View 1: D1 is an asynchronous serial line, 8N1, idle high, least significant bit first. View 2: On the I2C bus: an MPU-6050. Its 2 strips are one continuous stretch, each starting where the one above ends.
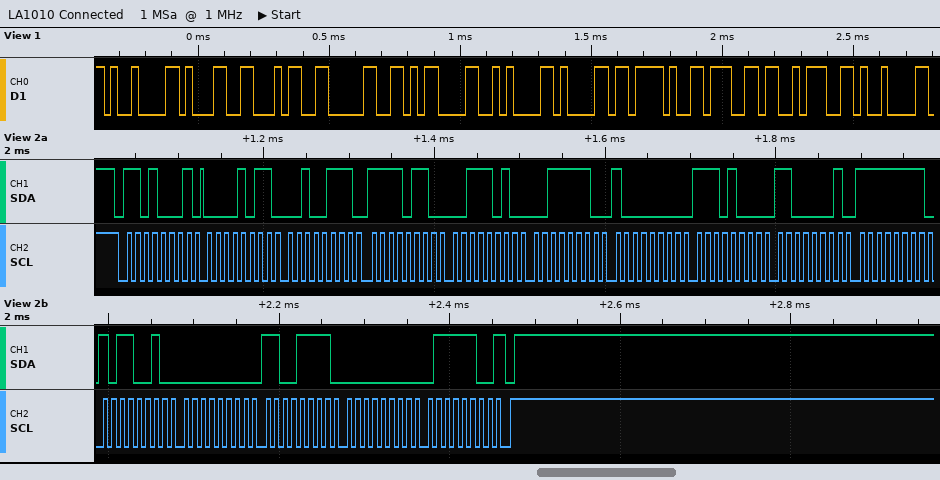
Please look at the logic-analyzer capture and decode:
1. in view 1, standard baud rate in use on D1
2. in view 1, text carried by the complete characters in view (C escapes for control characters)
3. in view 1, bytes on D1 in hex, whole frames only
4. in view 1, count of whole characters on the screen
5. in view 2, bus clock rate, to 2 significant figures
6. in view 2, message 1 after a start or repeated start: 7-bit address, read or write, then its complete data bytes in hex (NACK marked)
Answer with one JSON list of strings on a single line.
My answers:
["38400 baud", "\"\\t140\\r\\na/g:\\t\"", "0x09 0x31 0x34 0x30 0x0D 0x0A 0x61 0x2F 0x67 0x3A 0x09", "11", "100 kHz", "0x68 read: 0B 27 F6 3A 3E 80 E8 C1 FF B2 00 CF 00 7C NACK"]
